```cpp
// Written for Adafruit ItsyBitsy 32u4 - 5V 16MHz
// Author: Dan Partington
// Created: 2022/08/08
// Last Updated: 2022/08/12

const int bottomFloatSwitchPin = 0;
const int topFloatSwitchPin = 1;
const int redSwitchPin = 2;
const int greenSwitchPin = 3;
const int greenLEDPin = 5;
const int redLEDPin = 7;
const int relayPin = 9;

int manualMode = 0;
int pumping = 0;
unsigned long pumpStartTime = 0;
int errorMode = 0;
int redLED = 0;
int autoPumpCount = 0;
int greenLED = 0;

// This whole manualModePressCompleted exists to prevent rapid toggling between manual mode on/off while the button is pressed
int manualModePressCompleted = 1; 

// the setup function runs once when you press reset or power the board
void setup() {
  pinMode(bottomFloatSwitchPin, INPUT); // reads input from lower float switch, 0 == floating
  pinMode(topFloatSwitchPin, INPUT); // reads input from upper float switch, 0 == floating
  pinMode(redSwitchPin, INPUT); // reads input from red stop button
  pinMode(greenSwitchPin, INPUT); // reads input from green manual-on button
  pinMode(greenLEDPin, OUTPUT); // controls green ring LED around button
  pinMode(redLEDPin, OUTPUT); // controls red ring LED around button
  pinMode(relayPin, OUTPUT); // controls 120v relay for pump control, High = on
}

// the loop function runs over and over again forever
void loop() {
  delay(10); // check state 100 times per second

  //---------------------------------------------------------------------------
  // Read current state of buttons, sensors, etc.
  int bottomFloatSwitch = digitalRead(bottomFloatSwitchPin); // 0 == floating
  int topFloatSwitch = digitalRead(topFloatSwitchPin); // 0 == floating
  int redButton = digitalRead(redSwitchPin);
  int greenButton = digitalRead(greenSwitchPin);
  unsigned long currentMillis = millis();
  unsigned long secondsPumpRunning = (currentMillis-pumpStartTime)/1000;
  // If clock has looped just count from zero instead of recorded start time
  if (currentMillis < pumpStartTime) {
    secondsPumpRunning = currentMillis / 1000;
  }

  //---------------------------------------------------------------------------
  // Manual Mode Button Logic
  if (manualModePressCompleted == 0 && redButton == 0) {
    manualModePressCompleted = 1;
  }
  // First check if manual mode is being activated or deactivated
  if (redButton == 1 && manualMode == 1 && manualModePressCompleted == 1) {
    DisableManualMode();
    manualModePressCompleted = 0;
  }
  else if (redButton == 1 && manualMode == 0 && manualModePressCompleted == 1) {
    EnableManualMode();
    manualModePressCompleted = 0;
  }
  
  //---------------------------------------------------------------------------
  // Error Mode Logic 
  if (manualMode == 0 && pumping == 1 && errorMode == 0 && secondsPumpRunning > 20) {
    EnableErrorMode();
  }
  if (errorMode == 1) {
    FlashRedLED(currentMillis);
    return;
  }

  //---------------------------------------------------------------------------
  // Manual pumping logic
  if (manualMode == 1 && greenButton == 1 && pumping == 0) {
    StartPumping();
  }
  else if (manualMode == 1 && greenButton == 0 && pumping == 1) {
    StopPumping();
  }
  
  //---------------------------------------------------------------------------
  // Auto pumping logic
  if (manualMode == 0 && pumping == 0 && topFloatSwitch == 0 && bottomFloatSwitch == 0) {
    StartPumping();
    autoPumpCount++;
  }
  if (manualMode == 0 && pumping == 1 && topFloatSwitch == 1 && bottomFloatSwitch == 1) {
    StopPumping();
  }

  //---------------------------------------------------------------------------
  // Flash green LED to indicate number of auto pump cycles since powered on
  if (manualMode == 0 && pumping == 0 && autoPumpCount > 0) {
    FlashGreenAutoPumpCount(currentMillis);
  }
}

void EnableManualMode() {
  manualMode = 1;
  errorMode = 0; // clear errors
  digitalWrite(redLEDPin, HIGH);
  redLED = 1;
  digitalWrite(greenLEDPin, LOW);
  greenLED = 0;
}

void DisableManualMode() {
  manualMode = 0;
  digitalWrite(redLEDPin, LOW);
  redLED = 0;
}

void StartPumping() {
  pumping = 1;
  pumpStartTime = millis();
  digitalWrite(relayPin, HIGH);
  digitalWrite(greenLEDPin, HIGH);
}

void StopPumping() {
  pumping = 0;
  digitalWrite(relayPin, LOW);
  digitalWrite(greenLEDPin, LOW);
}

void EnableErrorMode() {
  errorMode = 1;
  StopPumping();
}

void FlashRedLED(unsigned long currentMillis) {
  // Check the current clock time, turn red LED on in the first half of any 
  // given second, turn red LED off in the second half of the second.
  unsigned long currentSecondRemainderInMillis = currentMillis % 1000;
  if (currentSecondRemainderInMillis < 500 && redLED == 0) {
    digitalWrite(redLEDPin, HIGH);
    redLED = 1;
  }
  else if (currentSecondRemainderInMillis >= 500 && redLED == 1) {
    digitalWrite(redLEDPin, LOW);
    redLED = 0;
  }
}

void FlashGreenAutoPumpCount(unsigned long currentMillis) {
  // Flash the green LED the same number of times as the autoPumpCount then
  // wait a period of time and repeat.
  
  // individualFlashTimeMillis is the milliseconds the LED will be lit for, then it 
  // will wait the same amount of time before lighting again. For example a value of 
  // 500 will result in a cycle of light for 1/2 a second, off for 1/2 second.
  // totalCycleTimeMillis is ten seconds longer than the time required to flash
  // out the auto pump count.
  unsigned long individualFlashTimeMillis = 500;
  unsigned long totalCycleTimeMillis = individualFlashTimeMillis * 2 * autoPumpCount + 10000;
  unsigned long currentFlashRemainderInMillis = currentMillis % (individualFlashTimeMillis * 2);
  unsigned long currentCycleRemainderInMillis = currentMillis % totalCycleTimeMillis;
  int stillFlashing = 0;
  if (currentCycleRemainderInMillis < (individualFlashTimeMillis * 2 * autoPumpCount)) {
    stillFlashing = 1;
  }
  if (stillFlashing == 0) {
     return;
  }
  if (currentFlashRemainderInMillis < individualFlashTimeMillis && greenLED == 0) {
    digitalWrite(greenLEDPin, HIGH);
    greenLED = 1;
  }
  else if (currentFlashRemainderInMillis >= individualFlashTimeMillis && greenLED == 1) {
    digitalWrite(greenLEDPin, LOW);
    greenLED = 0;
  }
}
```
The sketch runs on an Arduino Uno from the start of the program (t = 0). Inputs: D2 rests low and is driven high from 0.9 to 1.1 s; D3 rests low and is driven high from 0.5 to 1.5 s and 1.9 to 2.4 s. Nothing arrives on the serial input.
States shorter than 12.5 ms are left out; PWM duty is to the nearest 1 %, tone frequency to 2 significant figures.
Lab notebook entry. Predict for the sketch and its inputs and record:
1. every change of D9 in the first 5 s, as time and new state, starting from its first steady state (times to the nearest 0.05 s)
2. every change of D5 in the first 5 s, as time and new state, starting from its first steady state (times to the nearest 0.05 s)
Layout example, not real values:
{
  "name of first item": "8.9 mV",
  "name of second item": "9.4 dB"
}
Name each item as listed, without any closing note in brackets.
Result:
{
  "every change of D9 in the first 5 s, as time and new state, starting from its first steady state": "0 s high; 1.5 s low; 1.9 s high; 2.4 s low",
  "every change of D5 in the first 5 s, as time and new state, starting from its first steady state": "0 s high; 0.9 s low; 1.9 s high; 2.4 s low"
}
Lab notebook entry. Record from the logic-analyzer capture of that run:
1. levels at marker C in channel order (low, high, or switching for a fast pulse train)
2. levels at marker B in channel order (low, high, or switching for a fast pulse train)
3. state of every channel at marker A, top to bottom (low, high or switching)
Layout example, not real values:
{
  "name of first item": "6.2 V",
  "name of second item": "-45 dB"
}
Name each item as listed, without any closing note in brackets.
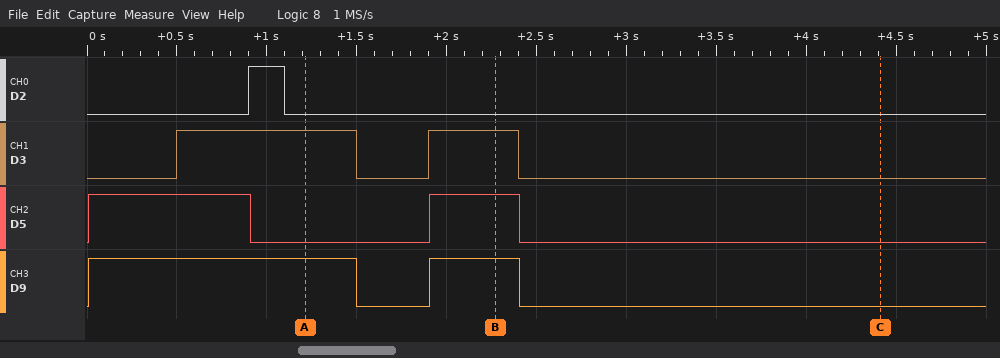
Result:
{
  "levels at marker C in channel order": "D2 low, D3 low, D5 low, D9 low",
  "levels at marker B in channel order": "D2 low, D3 high, D5 high, D9 high",
  "state of every channel at marker A, top to bottom": "D2 low, D3 high, D5 low, D9 high"
}
